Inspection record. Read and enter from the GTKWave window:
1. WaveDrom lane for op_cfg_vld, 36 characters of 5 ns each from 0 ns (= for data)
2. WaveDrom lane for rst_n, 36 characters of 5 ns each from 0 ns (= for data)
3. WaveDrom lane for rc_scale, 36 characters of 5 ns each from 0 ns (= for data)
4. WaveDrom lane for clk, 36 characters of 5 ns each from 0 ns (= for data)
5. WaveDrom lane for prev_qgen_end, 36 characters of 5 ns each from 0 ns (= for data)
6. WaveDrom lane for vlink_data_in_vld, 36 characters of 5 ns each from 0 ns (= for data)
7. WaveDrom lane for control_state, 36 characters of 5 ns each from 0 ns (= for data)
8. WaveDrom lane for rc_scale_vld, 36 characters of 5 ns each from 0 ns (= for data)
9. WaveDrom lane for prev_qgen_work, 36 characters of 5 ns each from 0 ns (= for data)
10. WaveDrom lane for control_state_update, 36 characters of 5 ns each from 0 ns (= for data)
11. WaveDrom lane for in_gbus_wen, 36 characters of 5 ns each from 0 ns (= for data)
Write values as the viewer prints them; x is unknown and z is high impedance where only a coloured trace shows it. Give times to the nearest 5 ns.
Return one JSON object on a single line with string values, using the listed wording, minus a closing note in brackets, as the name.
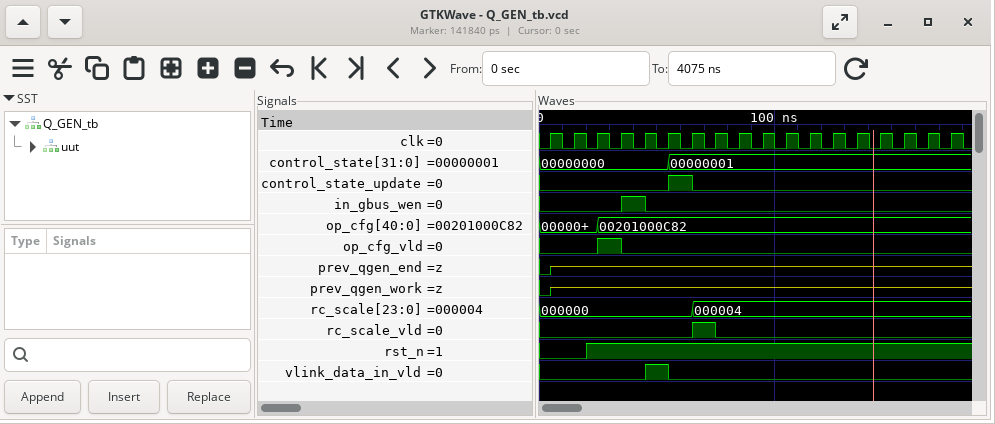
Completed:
{"WaveDrom lane for op_cfg_vld, 36 characters of 5 ns each from 0 ns": "{name: 'op_cfg_vld', wave: '0....1.0............................'}", "WaveDrom lane for rst_n, 36 characters of 5 ns each from 0 ns": "{name: 'rst_n', wave: '0...1...............................'}", "WaveDrom lane for rc_scale, 36 characters of 5 ns each from 0 ns": "{name: 'rc_scale', wave: '=............=......................', data: '000000 000004'}", "WaveDrom lane for clk, 36 characters of 5 ns each from 0 ns": "{name: 'clk', wave: '010101010101010101010101010101010101'}", "WaveDrom lane for prev_qgen_end, 36 characters of 5 ns each from 0 ns": "{name: 'prev_qgen_end', wave: '0z..................................'}", "WaveDrom lane for vlink_data_in_vld, 36 characters of 5 ns each from 0 ns": "{name: 'vlink_data_in_vld', wave: '0........1.0........................'}", "WaveDrom lane for control_state, 36 characters of 5 ns each from 0 ns": "{name: 'control_state', wave: '=..........=........................', data: '00000000 00000001'}", "WaveDrom lane for rc_scale_vld, 36 characters of 5 ns each from 0 ns": "{name: 'rc_scale_vld', wave: '0............1.0....................'}", "WaveDrom lane for prev_qgen_work, 36 characters of 5 ns each from 0 ns": "{name: 'prev_qgen_work', wave: '0z..................................'}", "WaveDrom lane for control_state_update, 36 characters of 5 ns each from 0 ns": "{name: 'control_state_update', wave: '0..........1.0......................'}", "WaveDrom lane for in_gbus_wen, 36 characters of 5 ns each from 0 ns": "{name: 'in_gbus_wen', wave: '0......1.0..........................'}"}
